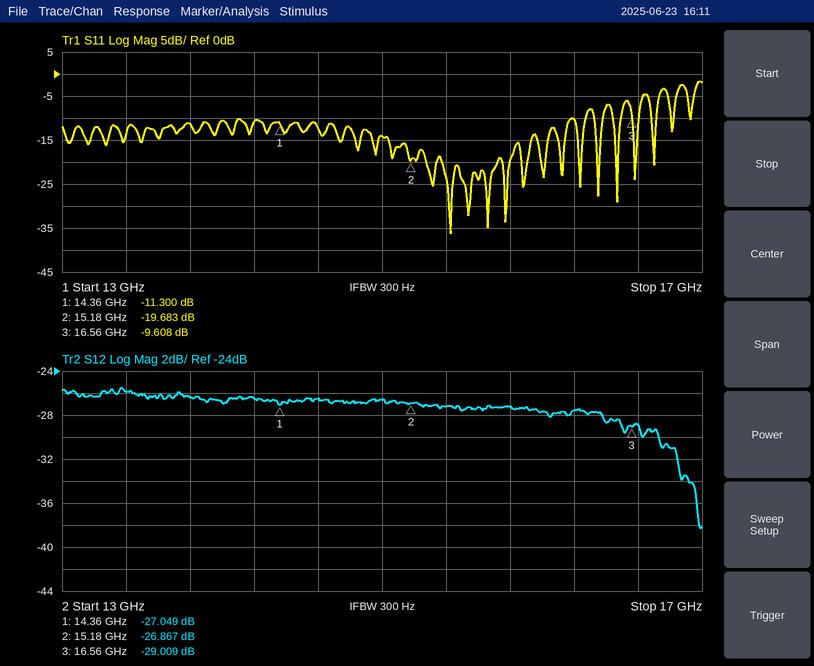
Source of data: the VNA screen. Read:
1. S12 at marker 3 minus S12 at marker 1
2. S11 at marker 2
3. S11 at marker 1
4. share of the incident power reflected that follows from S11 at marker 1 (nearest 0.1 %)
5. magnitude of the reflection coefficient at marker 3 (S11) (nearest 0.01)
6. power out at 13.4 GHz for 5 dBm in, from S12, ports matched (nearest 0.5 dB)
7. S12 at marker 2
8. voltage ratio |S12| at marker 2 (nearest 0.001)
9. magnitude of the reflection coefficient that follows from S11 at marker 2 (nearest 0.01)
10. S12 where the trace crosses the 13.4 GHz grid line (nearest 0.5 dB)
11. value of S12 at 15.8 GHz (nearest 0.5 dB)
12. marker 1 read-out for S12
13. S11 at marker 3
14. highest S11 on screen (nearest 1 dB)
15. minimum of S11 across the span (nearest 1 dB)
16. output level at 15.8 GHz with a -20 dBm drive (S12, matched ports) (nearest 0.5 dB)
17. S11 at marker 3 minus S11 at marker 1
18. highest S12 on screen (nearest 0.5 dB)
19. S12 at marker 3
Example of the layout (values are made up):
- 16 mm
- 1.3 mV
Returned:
- -1.960 dB
- -19.683 dB
- -11.300 dB
- 7.4 %
- 0.33
- -21.0 dBm
- -26.867 dB
- 0.045
- 0.10
- -26.0 dB
- -27.0 dB
- -27.049 dB
- -9.608 dB
- -2 dB
- -36 dB
- -47.0 dBm
- 1.692 dB
- -25.5 dB
- -29.009 dB
